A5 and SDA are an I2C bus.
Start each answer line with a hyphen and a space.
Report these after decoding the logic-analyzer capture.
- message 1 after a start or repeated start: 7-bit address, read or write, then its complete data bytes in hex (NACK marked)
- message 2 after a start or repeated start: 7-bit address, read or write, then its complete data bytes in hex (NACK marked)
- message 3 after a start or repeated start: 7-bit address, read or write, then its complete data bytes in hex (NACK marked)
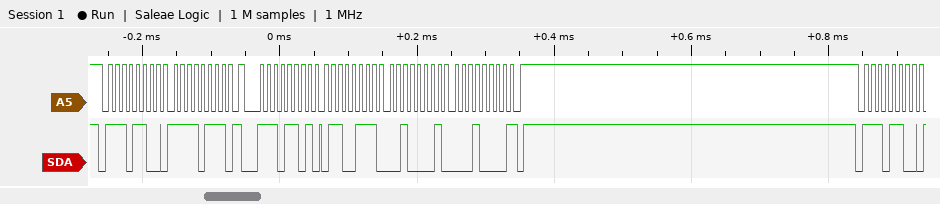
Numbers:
- 0x76 write: F7
- 0x76 read: 67 21 10 NACK
- 0x76 write
